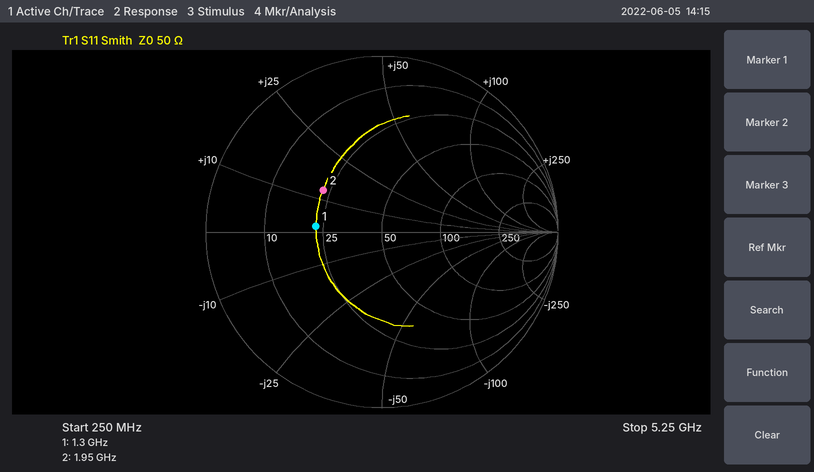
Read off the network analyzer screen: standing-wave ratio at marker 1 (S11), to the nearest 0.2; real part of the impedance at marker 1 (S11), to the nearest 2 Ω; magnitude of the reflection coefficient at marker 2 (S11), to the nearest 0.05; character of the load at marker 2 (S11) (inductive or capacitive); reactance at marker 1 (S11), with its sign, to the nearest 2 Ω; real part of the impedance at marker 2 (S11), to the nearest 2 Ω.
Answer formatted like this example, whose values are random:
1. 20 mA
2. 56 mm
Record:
1. 2.2
2. 22 Ω
3. 0.40
4. inductive
5. +2 Ω
6. 22 Ω
